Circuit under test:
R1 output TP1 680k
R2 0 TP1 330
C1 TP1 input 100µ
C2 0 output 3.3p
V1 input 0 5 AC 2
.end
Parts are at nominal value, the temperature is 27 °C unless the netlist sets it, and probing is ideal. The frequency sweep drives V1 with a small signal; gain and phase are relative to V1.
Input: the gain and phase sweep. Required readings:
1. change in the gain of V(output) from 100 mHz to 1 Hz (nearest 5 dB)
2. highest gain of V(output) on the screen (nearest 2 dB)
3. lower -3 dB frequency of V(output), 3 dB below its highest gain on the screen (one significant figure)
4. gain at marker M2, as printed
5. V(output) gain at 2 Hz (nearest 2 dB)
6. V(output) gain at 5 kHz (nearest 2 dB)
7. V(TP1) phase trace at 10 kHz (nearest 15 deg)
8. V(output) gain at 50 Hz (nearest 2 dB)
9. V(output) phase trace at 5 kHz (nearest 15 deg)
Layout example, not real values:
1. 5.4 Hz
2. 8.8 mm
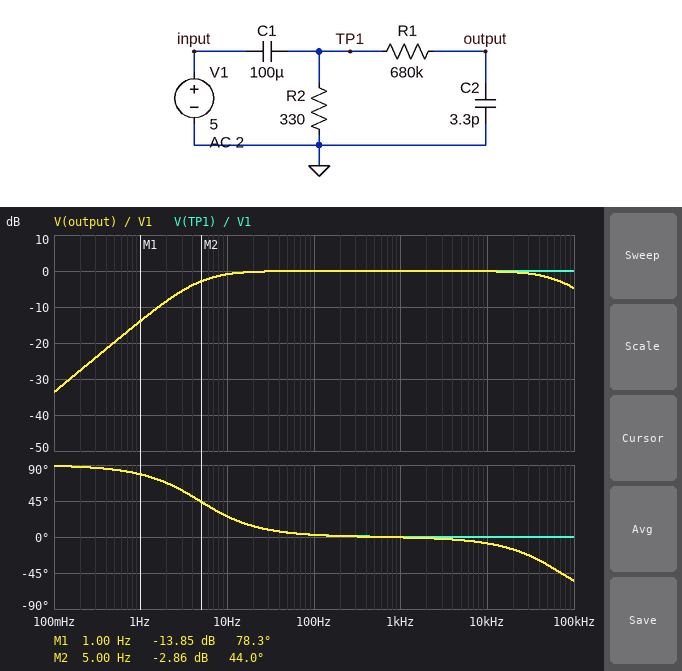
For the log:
1. 20 dB
2. 0 dB
3. 5 Hz
4. -2.86 dB
5. -8 dB
6. 0 dB
7. 0 deg
8. 0 dB
9. 0 deg
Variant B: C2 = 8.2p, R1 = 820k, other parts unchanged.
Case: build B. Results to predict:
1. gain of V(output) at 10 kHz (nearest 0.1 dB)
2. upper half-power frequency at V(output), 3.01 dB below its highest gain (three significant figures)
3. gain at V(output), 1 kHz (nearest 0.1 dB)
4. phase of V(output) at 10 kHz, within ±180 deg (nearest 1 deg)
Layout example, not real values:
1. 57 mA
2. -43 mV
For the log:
1. -0.7 dB
2. 23.7 kHz
3. 0 dB
4. -23 deg
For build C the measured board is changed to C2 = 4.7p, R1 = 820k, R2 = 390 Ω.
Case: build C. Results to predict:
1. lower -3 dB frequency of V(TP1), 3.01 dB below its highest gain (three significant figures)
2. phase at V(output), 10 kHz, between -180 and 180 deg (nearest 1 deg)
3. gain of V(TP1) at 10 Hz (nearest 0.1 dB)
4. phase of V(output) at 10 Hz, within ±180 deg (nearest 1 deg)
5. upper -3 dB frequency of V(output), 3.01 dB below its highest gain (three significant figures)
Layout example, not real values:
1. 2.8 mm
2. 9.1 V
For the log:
1. 4.08 Hz
2. -14 deg
3. -0.7 dB
4. 22 deg
5. 41.3 kHz
